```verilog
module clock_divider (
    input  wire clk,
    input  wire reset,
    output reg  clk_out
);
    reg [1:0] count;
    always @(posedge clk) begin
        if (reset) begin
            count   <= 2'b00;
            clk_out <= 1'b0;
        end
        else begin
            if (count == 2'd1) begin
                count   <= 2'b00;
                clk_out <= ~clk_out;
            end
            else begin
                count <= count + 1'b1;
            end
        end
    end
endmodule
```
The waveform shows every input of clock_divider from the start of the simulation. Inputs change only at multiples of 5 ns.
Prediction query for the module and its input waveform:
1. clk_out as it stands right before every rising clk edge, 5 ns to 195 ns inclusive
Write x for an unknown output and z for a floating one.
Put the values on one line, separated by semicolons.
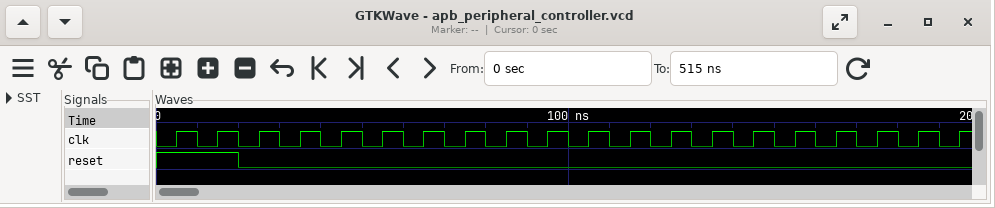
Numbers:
x 0 0 0 1 1 0 0 1 1 0 0 1 1 0 0 1 1 0 0
